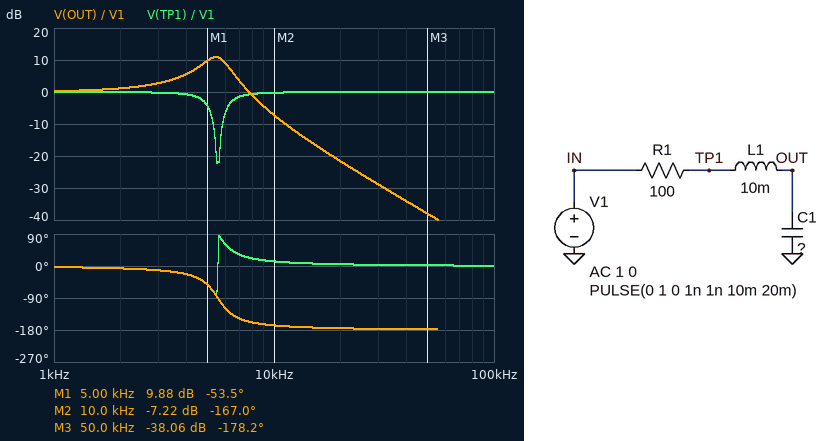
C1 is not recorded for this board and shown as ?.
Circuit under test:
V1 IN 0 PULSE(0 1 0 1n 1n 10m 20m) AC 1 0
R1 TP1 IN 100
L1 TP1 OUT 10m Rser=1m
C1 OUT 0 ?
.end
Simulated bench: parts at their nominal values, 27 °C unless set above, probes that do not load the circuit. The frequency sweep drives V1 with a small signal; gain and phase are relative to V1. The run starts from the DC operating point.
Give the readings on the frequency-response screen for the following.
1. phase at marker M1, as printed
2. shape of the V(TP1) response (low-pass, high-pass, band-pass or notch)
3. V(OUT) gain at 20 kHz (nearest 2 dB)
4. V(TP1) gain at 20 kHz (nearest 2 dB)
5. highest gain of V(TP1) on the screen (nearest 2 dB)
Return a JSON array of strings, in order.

["-53.5 deg", "notch", "-22 dB", "0 dB", "0 dB"]
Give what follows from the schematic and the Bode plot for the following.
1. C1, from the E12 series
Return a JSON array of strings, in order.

["82 nF"]
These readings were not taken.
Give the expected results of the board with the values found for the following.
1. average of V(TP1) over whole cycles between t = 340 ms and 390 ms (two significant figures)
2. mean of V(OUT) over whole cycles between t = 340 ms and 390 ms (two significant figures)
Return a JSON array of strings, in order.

["500 mV", "500 mV"]
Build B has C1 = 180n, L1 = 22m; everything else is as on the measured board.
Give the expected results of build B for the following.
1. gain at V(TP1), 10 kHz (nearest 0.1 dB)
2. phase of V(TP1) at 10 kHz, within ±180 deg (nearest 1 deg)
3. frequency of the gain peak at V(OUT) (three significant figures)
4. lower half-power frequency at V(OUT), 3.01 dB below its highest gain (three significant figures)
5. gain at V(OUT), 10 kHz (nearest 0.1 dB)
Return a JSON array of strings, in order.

["0 dB", "4 deg", "2.48 kHz", "2.08 kHz", "-23.3 dB"]
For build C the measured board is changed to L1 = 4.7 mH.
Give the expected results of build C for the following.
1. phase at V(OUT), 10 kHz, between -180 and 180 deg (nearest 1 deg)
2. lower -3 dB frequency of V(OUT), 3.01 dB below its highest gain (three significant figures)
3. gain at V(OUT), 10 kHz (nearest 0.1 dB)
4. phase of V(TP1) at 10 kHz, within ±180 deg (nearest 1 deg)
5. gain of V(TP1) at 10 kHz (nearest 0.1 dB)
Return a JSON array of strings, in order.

["-135 deg", "5.76 kHz", "2.7 dB", "45 deg", "-3.0 dB"]
